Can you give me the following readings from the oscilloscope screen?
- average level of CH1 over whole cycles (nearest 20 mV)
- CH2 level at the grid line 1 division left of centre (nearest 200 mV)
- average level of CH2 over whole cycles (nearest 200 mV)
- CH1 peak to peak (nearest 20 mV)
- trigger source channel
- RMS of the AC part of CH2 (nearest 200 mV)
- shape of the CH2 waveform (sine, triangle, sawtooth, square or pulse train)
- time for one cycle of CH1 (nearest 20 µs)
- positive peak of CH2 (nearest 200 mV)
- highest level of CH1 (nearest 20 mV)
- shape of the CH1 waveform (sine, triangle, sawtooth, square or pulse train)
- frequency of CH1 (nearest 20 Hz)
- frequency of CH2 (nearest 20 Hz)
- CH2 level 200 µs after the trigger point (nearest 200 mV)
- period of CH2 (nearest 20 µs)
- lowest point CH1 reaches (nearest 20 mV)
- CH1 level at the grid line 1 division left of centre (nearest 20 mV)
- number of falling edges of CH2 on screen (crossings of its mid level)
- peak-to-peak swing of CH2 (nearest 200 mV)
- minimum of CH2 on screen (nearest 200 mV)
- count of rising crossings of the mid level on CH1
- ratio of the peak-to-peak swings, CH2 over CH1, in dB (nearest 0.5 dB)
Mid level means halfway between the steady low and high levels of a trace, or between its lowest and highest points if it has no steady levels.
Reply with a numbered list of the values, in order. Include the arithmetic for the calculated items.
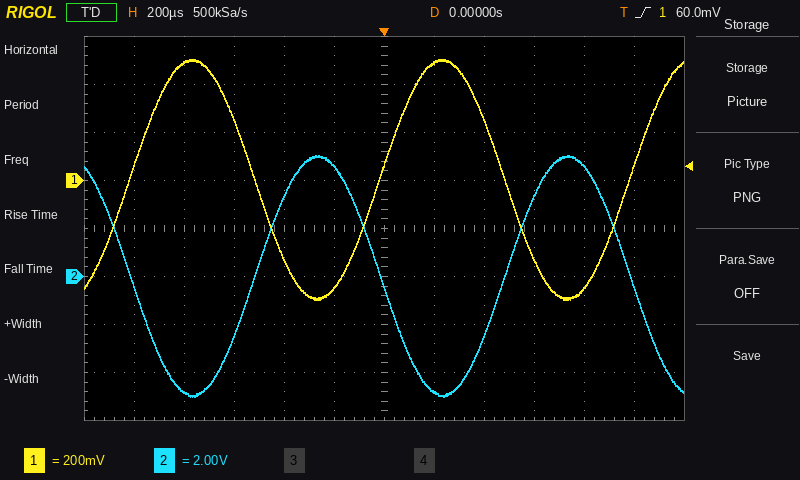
1. (500 mV + (-500 mV)) / 2 ≈ 0 mV
2. 4.6 V
3. (5.0 V + (-5.0 V)) / 2 ≈ 0.0 V
4. 500 mV − (-500 mV) = 1.00 V
5. CH1
6. 10.0 V / (2√2) ≈ 3.54 V, so 3.6 V to the nearest 200 mV
7. sine
8. 1.00 ms
9. 5.0 V
10. 500 mV
11. sine
12. 1 / 1.00 ms ≈ 1.00 kHz
13. 1 / 1.00 ms ≈ 1.00 kHz
14. -4.8 V
15. 1.00 ms
16. -500 mV
17. -440 mV
18. 3
19. 5.0 V − (-5.0 V) = 10.0 V
20. -5.0 V
21. 3
22. 20 log10(10.0 V / 1.00 V) ≈ 20.0 dB
